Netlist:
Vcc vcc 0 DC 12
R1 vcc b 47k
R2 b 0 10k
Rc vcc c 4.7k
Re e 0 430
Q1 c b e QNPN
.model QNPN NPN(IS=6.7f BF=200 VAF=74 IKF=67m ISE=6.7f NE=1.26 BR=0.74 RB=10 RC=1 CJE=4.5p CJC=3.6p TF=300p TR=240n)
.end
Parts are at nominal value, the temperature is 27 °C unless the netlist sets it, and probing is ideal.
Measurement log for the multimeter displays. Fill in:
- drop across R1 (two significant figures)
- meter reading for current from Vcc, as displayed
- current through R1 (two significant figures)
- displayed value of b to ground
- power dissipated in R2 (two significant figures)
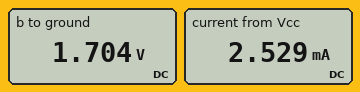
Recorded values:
10 V
2.529 mA
220 µA
1.704 V
290 µW
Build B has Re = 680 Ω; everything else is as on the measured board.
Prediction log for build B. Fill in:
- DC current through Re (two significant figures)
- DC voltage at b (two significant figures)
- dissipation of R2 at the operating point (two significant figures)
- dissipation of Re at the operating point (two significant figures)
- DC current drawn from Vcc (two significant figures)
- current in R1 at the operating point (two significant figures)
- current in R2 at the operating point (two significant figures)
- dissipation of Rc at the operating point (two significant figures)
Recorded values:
1.9 mA
2.0 V
380 µW
2.4 mW
2.1 mA
210 µA
200 µA
16 mW
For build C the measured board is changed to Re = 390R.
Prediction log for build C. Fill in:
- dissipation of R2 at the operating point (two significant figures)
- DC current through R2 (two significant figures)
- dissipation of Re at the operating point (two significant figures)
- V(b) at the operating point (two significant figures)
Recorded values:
260 µW
160 µA
2.2 mW
1.6 V
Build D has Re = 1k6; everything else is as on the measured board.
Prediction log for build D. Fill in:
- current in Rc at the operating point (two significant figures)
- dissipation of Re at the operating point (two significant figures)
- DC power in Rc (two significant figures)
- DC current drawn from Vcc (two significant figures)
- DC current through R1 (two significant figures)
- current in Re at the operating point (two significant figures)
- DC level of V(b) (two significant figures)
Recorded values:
850 µA
1.2 mW
3.4 mW
1.1 mA
210 µA
860 µA
2.0 V
